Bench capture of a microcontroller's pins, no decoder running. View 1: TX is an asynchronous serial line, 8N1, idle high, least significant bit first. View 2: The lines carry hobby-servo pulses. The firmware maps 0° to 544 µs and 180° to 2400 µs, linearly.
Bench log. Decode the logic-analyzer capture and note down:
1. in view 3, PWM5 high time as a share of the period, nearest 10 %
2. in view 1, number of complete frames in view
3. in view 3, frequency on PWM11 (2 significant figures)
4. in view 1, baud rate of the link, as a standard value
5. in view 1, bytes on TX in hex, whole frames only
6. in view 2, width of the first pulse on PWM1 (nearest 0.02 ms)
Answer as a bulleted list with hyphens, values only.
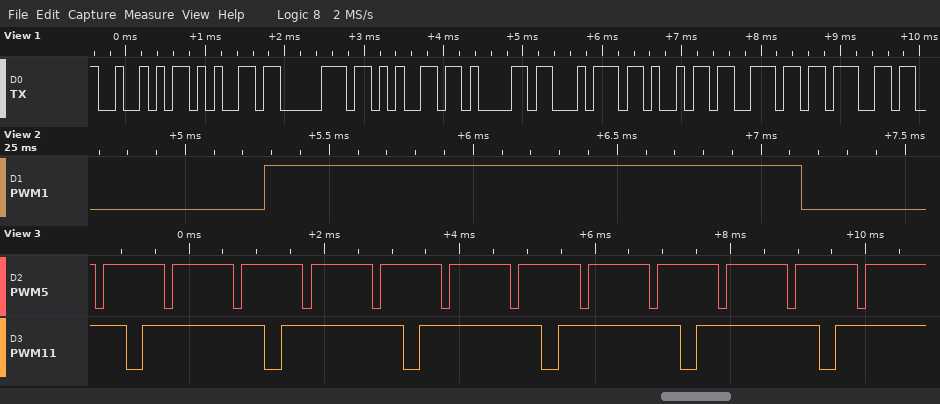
- 90 %
- 9
- 490 Hz
- 9600 baud
- 0x52 0x65 0x70 0x65 0x61 0x74 0x69 0x6E 0x67
- 1.86 ms
